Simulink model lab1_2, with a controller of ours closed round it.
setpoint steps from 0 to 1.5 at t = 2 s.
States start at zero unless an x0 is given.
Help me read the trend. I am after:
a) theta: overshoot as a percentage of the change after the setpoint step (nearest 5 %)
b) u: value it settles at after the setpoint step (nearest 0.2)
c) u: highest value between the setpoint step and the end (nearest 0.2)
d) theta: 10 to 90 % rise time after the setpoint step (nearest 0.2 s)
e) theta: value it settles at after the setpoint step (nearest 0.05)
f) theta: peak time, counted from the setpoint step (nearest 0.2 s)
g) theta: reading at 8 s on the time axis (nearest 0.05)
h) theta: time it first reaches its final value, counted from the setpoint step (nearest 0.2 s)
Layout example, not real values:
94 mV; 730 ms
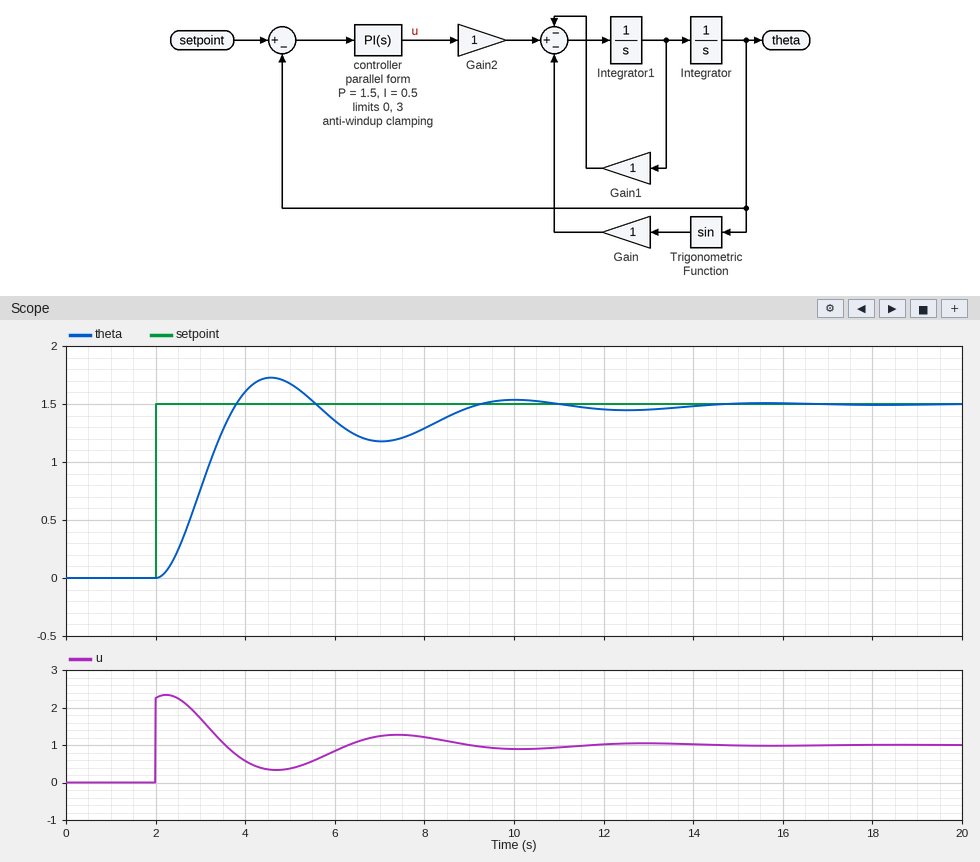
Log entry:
15 %; 1.0; 2.4; 1.2 s; 1.50; 2.6 s; 1.30; 1.8 s
